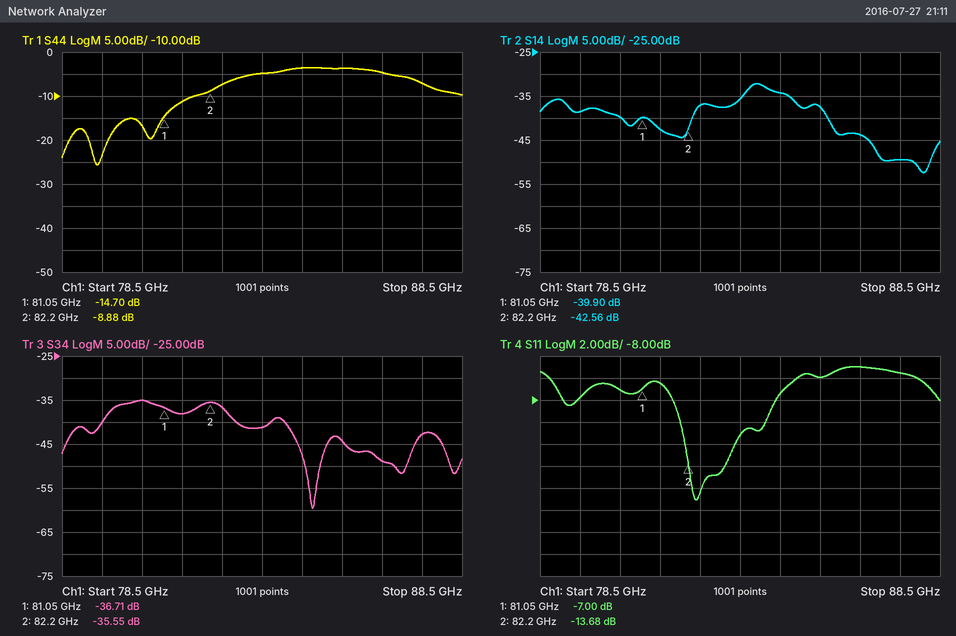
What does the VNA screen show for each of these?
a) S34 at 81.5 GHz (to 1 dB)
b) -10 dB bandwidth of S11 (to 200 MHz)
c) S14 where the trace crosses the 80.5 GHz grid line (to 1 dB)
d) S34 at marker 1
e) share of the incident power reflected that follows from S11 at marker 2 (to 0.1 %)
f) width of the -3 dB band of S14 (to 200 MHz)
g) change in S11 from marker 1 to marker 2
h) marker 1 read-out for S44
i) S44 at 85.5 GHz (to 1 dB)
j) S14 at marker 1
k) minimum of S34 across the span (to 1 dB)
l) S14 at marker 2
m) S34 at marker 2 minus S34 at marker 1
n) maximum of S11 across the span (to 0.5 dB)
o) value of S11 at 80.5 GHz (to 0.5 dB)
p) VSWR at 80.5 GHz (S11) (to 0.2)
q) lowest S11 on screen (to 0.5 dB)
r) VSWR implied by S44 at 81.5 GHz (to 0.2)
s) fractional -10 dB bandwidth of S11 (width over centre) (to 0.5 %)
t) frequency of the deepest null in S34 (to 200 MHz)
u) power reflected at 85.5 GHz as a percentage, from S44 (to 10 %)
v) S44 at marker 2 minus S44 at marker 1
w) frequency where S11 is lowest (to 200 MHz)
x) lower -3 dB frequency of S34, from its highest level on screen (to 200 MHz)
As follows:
-38 dB
2.2 GHz
-40 dB
-36.71 dB
4.3 %
1.2 GHz
-6.68 dB
-14.70 dB
-4 dB
-39.90 dB
-60 dB
-42.56 dB
1.16 dB
-5.0 dB
-7.0 dB
2.6
-17.0 dB
1.8
2.5 %
84.8 GHz
40 %
5.82 dB
82.4 GHz
79.6 GHz
